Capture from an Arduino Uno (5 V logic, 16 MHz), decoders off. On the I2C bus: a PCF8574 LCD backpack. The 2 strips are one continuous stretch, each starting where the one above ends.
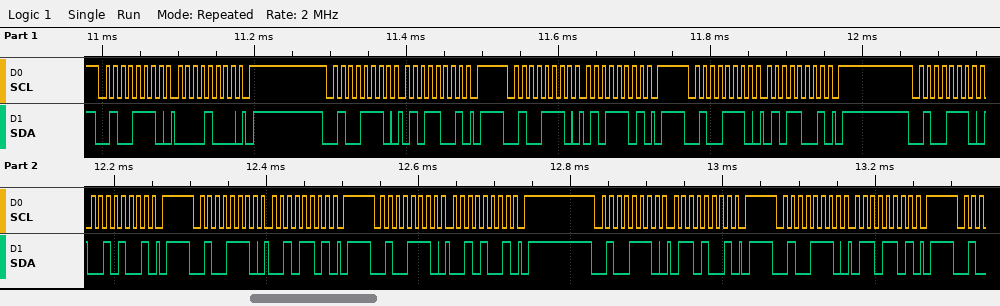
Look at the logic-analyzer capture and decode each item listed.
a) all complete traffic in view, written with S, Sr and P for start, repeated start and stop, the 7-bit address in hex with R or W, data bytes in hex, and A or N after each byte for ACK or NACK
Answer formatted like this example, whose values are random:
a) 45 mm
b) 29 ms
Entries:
a) S 27W A 08 A P S 27W A 59 A P S 27W A 5D A P S 27W A 59 A P S 27W A 29 A P S 27W A 2D A P S 27W A 29 A P S 27W A 69 A P S 27W A 6D A P
